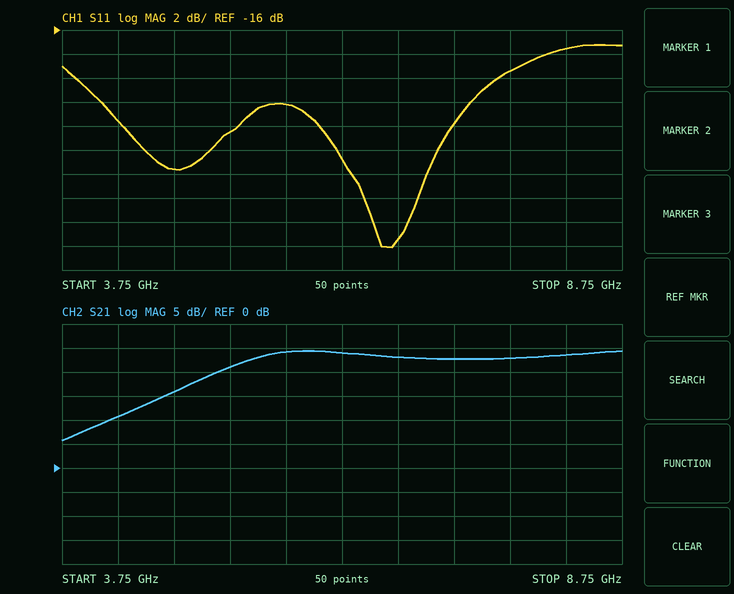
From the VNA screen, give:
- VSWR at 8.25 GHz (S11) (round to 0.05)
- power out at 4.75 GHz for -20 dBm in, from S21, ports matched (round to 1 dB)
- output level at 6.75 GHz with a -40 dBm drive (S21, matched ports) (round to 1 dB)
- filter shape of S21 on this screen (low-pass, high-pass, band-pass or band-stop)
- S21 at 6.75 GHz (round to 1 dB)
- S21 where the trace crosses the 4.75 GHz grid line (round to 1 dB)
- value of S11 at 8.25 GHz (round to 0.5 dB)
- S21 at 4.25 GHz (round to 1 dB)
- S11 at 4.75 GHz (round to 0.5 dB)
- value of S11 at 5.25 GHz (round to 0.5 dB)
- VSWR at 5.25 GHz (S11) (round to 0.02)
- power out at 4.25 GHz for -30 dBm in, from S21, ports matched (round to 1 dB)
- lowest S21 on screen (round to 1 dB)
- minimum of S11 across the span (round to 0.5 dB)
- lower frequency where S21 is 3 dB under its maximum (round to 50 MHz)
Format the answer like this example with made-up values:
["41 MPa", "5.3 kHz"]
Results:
["1.30", "-4 dBm", "-17 dBm", "high-pass", "23 dB", "16 dB", "-17.5 dB", "11 dB", "-27.5 dB", "-24.5 dB", "1.12", "-19 dBm", "6 dB", "-34.0 dB", "5.30 GHz"]
